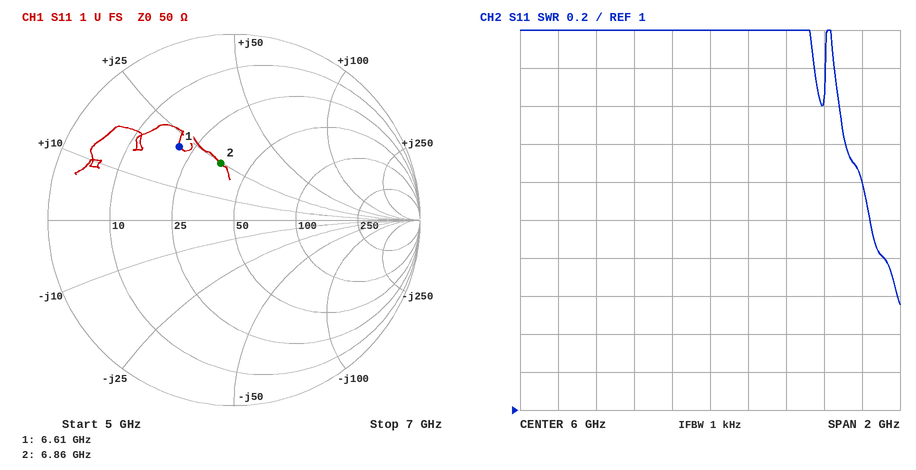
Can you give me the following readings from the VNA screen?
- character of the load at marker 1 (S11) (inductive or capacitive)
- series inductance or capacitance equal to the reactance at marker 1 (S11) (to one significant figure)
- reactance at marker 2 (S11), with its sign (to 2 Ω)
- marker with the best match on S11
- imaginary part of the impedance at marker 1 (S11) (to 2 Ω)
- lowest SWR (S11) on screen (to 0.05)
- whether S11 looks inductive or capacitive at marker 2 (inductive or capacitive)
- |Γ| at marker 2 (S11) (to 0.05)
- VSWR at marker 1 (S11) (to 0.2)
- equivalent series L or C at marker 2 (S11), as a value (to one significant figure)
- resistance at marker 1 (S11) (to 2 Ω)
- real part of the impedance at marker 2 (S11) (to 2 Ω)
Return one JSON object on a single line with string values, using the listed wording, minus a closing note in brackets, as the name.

{"character of the load at marker 1 (S11)": "inductive", "series inductance or capacitance equal to the reactance at marker 1 (S11)": "500 pH", "reactance at marker 2 (S11), with its sign": "+24 Ω", "marker with the best match on S11": "marker 2", "imaginary part of the impedance at marker 1 (S11)": "+22 Ω", "lowest SWR (S11) on screen": "1.55", "whether S11 looks inductive or capacitive at marker 2": "inductive", "|Γ| at marker 2 (S11)": "0.30", "VSWR at marker 1 (S11)": "3.0", "equivalent series L or C at marker 2 (S11), as a value": "600 pH", "resistance at marker 1 (S11)": "20 Ω", "real part of the impedance at marker 2 (S11)": "36 Ω"}
